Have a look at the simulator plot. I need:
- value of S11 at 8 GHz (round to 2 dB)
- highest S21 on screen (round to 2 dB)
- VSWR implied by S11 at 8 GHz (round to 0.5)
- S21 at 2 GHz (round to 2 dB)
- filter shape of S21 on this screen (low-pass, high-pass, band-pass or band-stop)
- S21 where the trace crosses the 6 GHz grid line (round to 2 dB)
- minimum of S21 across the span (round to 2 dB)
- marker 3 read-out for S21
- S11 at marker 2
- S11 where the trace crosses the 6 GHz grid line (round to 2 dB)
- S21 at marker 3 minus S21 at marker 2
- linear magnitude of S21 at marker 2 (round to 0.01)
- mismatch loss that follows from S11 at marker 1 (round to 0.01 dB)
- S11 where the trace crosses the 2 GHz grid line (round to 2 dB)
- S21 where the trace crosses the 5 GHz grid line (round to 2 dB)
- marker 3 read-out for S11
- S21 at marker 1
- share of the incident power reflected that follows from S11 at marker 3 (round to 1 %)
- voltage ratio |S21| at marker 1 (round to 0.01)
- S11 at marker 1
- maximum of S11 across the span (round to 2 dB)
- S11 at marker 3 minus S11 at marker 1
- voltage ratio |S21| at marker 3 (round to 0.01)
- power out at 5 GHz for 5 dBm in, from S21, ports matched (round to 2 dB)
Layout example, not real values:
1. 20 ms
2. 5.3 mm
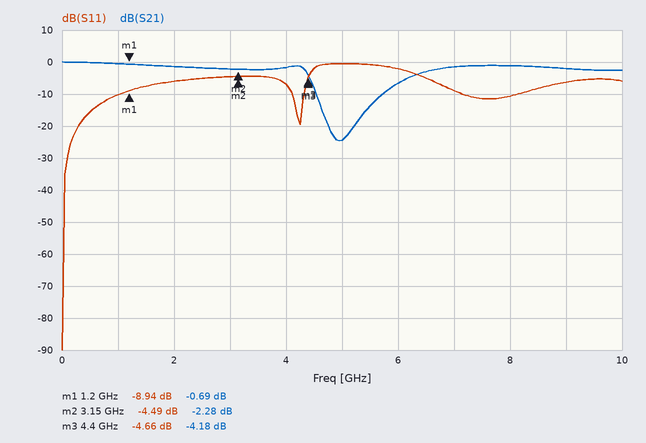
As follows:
1. -10 dB
2. 0 dB
3. 2.0
4. -2 dB
5. band-stop
6. -6 dB
7. -24 dB
8. -4.18 dB
9. -4.49 dB
10. -2 dB
11. -1.90 dB
12. 0.77
13. 0.59 dB
14. -6 dB
15. -24 dB
16. -4.66 dB
17. -0.69 dB
18. 34 %
19. 0.92
20. -8.94 dB
21. 0 dB
22. 4.28 dB
23. 0.62
24. -20 dBm
